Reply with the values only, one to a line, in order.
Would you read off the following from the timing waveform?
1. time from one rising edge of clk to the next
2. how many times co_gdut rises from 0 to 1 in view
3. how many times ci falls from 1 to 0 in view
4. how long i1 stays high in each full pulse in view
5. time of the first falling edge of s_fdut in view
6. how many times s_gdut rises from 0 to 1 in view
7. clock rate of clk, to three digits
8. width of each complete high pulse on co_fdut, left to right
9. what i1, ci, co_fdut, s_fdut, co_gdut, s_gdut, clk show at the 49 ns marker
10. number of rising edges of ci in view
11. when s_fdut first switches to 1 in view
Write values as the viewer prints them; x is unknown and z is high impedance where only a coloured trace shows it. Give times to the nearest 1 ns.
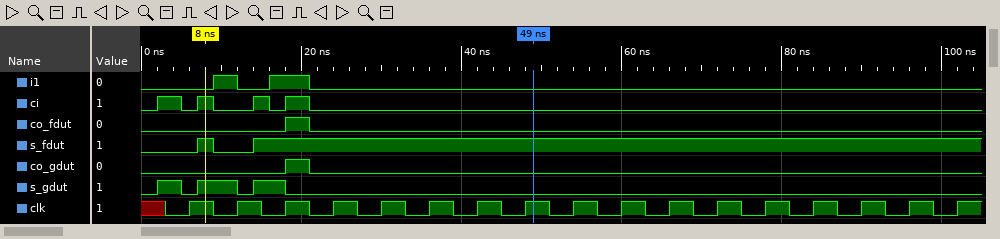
6 ns
1
4
3 ns, 5 ns
9 ns
3
167 MHz
3 ns
i1=0, ci=0, co_fdut=0, s_fdut=1, co_gdut=0, s_gdut=0, clk=1
4
7 ns
